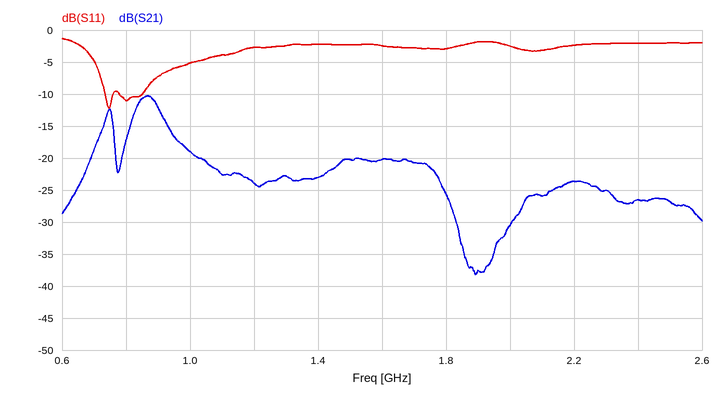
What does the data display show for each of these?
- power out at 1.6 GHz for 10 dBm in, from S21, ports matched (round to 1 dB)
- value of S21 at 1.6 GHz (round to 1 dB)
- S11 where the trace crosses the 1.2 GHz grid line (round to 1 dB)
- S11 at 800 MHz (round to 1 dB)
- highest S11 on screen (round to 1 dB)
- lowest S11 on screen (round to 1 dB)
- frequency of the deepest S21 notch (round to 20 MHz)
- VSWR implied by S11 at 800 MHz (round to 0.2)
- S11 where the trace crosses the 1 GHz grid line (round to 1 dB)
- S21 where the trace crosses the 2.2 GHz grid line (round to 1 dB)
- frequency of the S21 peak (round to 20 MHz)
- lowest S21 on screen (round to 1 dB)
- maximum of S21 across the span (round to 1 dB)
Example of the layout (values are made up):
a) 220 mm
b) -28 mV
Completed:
a) -10 dBm
b) -20 dB
c) -3 dB
d) -11 dB
e) -1 dB
f) -12 dB
g) 1.90 GHz
h) 1.8
i) -5 dB
j) -24 dB
k) 860 MHz
l) -38 dB
m) -10 dB
